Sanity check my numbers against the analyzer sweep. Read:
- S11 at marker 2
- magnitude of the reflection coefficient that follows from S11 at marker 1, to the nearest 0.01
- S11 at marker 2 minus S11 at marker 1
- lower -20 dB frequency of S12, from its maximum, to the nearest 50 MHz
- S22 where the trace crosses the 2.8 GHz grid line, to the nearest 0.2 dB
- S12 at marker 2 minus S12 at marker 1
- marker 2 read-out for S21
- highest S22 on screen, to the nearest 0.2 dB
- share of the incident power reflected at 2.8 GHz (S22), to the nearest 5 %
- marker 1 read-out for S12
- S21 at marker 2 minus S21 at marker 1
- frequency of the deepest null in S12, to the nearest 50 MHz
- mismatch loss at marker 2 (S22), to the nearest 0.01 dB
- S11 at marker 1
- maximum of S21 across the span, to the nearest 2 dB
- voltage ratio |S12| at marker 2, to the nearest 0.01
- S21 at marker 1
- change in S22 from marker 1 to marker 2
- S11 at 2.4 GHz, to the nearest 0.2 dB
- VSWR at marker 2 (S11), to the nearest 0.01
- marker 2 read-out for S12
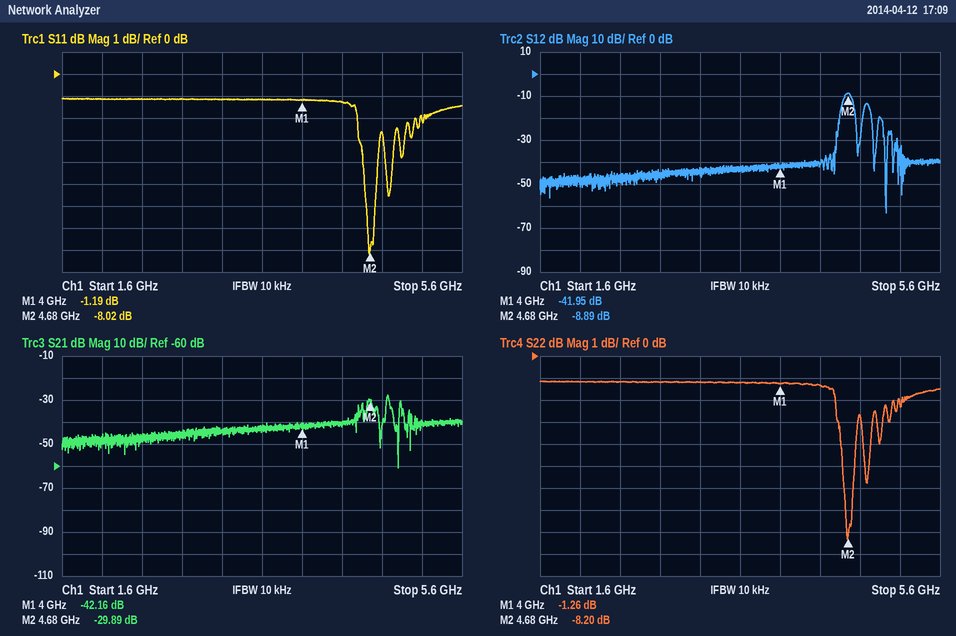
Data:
-8.02 dB
0.87
-6.83 dB
4.55 GHz
-1.2 dB
33.06 dB
-29.89 dB
-1.2 dB
75 %
-41.95 dB
12.27 dB
5.05 GHz
0.71 dB
-1.19 dB
-28 dB
0.36
-42.16 dB
-6.94 dB
-1.2 dB
2.32
-8.89 dB
